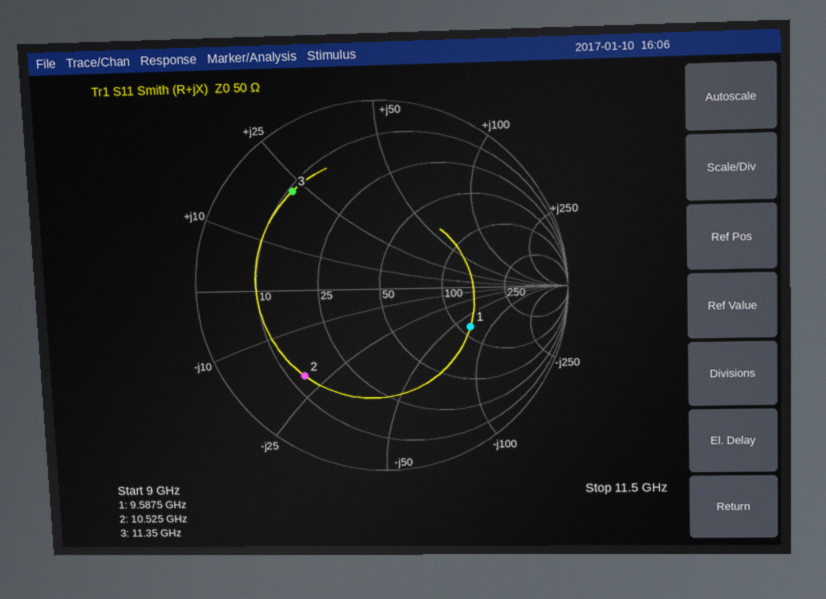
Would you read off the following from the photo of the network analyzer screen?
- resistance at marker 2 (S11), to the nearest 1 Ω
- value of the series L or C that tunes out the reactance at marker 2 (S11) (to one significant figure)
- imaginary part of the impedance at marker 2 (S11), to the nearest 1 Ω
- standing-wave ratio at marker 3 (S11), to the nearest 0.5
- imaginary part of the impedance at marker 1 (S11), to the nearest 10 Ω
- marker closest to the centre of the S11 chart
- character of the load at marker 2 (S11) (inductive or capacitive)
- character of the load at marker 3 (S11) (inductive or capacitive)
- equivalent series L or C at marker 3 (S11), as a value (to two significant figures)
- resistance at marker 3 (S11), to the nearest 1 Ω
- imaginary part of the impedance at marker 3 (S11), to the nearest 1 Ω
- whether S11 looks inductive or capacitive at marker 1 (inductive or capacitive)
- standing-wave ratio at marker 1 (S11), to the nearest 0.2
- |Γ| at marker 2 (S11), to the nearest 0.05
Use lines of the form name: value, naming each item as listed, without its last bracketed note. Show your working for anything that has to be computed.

resistance at marker 2 (S11), to the nearest 1 Ω: 13 Ω
value of the series L or C that tunes out the reactance at marker 2 (S11): L = 21 Ω/(2π × 10.525 GHz) ≈ 318 pH, so 300 pH to one significant figure
imaginary part of the impedance at marker 2 (S11), to the nearest 1 Ω: -21 Ω
standing-wave ratio at marker 3 (S11), to the nearest 0.5: 5.5
imaginary part of the impedance at marker 1 (S11), to the nearest 10 Ω: -70 Ω
marker closest to the centre of the S11 chart: marker 1
character of the load at marker 2 (S11): capacitive
character of the load at marker 3 (S11): inductive
equivalent series L or C at marker 3 (S11), as a value: L = 22 Ω/(2π × 11.35 GHz) ≈ 308 pH, so 310 pH to two significant figures
resistance at marker 3 (S11), to the nearest 1 Ω: 11 Ω
imaginary part of the impedance at marker 3 (S11), to the nearest 1 Ω: +22 Ω
whether S11 looks inductive or capacitive at marker 1: capacitive
standing-wave ratio at marker 1 (S11), to the nearest 0.2: 3.2
|Γ| at marker 2 (S11), to the nearest 0.05: 0.65
